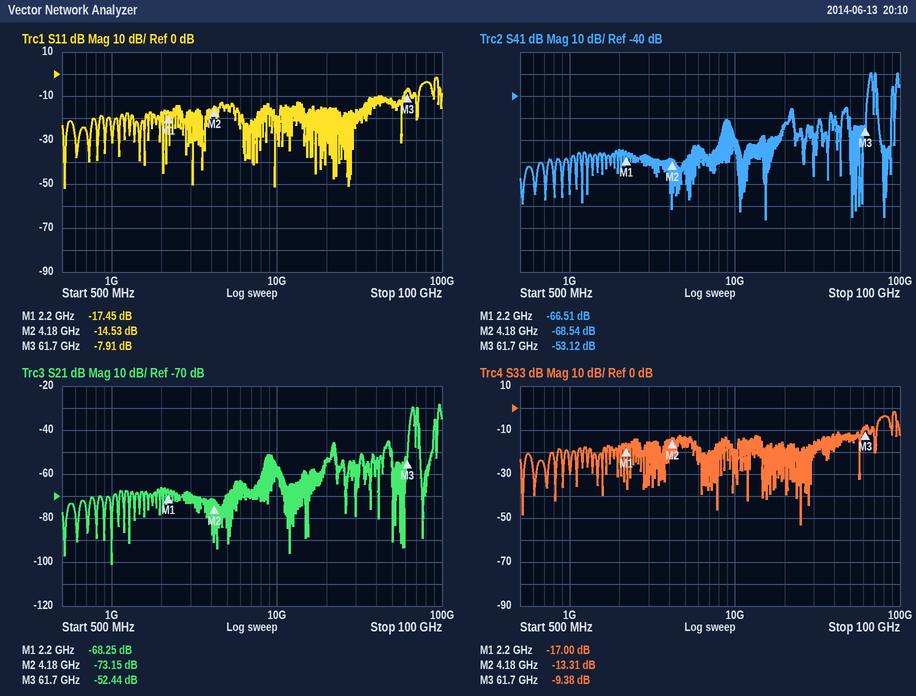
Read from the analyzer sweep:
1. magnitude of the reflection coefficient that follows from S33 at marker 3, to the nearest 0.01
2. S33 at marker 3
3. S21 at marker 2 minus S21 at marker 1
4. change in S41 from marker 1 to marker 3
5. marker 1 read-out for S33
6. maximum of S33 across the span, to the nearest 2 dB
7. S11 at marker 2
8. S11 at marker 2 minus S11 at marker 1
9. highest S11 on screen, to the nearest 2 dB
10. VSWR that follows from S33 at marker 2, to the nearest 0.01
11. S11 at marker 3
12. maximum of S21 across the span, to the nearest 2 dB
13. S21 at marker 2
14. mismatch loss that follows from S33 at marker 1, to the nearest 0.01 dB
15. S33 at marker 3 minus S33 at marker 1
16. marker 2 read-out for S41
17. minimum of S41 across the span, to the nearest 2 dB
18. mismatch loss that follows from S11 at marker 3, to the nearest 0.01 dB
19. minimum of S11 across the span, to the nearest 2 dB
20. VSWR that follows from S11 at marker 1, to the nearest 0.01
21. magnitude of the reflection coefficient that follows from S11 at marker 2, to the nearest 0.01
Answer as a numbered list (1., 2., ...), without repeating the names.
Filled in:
1. 0.34
2. -9.38 dB
3. -4.90 dB
4. 13.39 dB
5. -17.00 dB
6. -2 dB
7. -14.53 dB
8. 2.92 dB
9. -2 dB
10. 1.55
11. -7.91 dB
12. -28 dB
13. -73.15 dB
14. 0.09 dB
15. 7.62 dB
16. -68.54 dB
17. -96 dB
18. 0.77 dB
19. -52 dB
20. 1.31
21. 0.19
